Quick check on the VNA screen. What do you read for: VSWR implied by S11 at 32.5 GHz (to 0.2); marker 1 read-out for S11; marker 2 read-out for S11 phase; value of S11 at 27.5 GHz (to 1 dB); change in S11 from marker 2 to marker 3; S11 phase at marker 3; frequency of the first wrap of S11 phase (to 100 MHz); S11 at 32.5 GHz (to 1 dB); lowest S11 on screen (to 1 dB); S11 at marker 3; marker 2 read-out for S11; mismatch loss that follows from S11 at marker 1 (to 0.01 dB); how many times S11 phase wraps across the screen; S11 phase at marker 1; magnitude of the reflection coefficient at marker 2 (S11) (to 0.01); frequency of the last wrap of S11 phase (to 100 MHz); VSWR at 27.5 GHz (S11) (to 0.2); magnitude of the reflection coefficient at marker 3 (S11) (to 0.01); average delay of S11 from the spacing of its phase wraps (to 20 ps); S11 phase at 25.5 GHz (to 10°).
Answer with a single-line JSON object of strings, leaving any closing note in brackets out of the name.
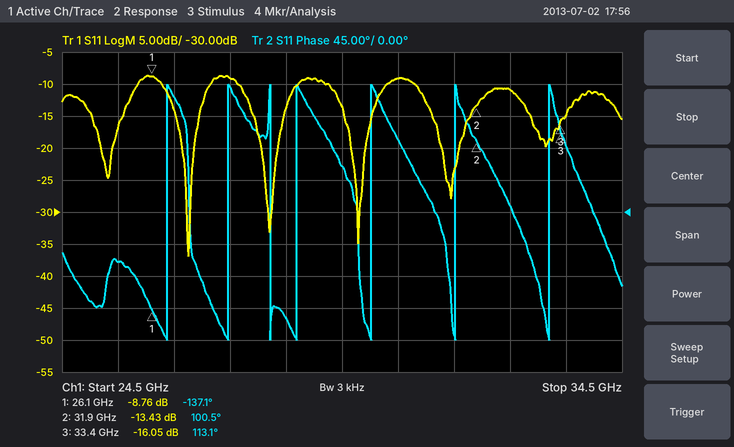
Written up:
{"VSWR implied by S11 at 32.5 GHz": "1.8", "marker 1 read-out for S11": "-8.76 dB", "marker 2 read-out for S11 phase": "100.5°", "value of S11 at 27.5 GHz": "-9 dB", "change in S11 from marker 2 to marker 3": "-2.62 dB", "S11 phase at marker 3": "113.1°", "frequency of the first wrap of S11 phase": "26.4 GHz", "S11 at 32.5 GHz": "-11 dB", "lowest S11 on screen": "-37 dB", "S11 at marker 3": "-16.05 dB", "marker 2 read-out for S11": "-13.43 dB", "mismatch loss that follows from S11 at marker 1": "0.62 dB", "how many times S11 phase wraps across the screen": "7", "S11 phase at marker 1": "-137.1°", "magnitude of the reflection coefficient at marker 2 (S11)": "0.21", "frequency of the last wrap of S11 phase": "33.2 GHz", "VSWR at 27.5 GHz (S11)": "2.0", "magnitude of the reflection coefficient at marker 3 (S11)": "0.16", "average delay of S11 from the spacing of its phase wraps": "880 ps", "S11 phase at 25.5 GHz": "-70°"}
